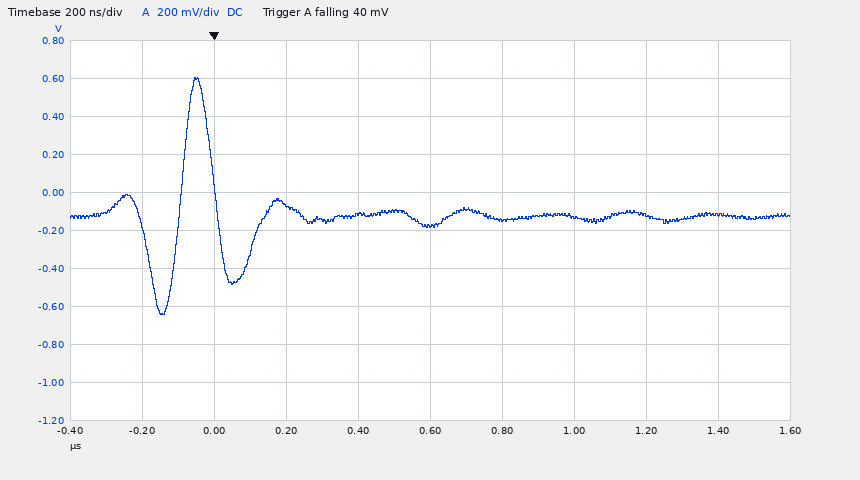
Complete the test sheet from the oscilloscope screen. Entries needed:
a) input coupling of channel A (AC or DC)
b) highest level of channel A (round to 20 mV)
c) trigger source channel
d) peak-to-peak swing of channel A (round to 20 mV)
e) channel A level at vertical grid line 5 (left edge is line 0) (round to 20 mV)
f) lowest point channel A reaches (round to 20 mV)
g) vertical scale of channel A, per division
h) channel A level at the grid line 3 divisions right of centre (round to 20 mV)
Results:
DC
600 mV
channel A
1.24 V
-180 mV
-640 mV
200 mV
-120 mV
